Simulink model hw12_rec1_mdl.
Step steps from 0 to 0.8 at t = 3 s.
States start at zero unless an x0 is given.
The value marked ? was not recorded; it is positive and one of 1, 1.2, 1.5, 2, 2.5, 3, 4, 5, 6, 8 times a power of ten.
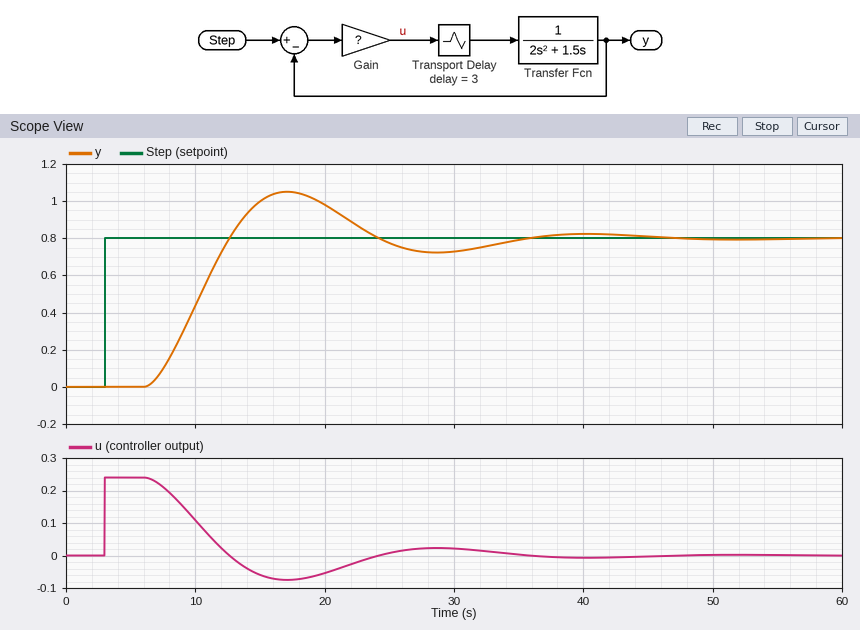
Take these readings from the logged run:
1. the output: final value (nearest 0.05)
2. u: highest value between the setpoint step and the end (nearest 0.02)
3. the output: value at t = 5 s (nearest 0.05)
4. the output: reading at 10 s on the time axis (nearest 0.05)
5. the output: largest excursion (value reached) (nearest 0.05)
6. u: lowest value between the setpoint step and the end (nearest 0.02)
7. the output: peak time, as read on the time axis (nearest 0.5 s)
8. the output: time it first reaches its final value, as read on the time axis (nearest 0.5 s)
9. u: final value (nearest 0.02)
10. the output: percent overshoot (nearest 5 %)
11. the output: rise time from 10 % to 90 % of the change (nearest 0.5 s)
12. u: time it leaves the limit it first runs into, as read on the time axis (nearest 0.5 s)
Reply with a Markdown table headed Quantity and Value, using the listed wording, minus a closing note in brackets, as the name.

| Quantity | Value |
|---|---|
| the output: final value | 0.80 |
| u: highest value between the setpoint step and the end | 0.24 |
| the output: value at t = 5 s | 0.00 |
| the output: reading at 10 s on the time axis | 0.45 |
| the output: largest excursion (value reached) | 1.05 |
| u: lowest value between the setpoint step and the end | -0.08 |
| the output: peak time, as read on the time axis | 17.0 s |
| the output: time it first reaches its final value, as read on the time axis | 12.5 s |
| u: final value | 0.00 |
| the output: percent overshoot | 30 % |
| the output: rise time from 10 % to 90 % of the change | 4.5 s |
| u: time it leaves the limit it first runs into, as read on the time axis | 6.5 s |
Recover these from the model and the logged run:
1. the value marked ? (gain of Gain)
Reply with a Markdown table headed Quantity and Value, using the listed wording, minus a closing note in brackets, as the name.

| Quantity | Value |
|---|---|
| the value marked ? | 0.3 |
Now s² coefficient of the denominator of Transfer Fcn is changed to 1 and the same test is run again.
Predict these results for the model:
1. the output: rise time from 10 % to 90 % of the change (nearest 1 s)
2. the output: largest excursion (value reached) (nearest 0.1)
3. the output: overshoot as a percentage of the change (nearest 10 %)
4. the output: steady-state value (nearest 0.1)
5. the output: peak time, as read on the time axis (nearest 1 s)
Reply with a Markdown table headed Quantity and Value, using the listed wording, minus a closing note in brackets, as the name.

| Quantity | Value |
|---|---|
| the output: rise time from 10 % to 90 % of the change | 4 s |
| the output: largest excursion (value reached) | 1.0 |
| the output: overshoot as a percentage of the change | 20 % |
| the output: steady-state value | 0.8 |
| the output: peak time, as read on the time axis | 16 s |
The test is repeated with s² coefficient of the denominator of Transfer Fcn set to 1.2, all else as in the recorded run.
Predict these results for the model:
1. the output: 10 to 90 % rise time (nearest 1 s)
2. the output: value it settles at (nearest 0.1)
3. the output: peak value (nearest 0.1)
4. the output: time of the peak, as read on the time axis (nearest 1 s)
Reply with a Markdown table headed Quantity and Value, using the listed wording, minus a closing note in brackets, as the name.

| Quantity | Value |
|---|---|
| the output: 10 to 90 % rise time | 4 s |
| the output: value it settles at | 0.8 |
| the output: peak value | 1.0 |
| the output: time of the peak, as read on the time axis | 16 s |
